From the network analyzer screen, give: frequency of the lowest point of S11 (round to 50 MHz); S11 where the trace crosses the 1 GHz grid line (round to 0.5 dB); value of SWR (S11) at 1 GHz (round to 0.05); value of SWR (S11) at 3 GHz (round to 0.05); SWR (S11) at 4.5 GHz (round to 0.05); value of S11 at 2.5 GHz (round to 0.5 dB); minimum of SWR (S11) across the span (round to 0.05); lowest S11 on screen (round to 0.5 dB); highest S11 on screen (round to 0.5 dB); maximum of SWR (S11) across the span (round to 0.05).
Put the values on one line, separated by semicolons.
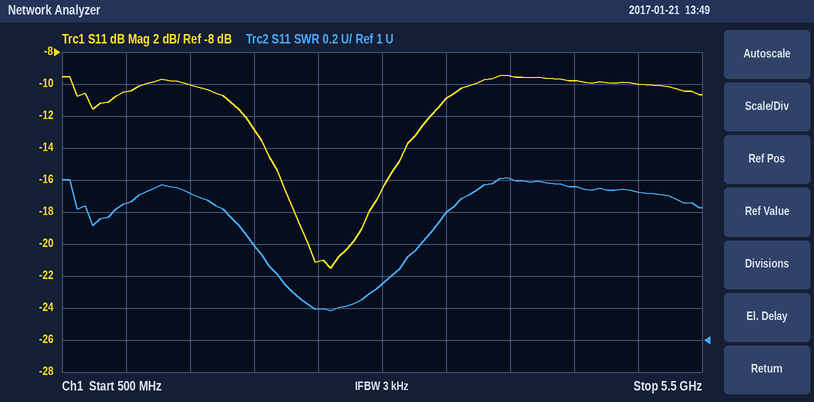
2.60 GHz; -10.5 dB; 1.85; 1.35; 1.95; -21.0 dB; 1.20; -21.5 dB; -9.5 dB; 2.00
